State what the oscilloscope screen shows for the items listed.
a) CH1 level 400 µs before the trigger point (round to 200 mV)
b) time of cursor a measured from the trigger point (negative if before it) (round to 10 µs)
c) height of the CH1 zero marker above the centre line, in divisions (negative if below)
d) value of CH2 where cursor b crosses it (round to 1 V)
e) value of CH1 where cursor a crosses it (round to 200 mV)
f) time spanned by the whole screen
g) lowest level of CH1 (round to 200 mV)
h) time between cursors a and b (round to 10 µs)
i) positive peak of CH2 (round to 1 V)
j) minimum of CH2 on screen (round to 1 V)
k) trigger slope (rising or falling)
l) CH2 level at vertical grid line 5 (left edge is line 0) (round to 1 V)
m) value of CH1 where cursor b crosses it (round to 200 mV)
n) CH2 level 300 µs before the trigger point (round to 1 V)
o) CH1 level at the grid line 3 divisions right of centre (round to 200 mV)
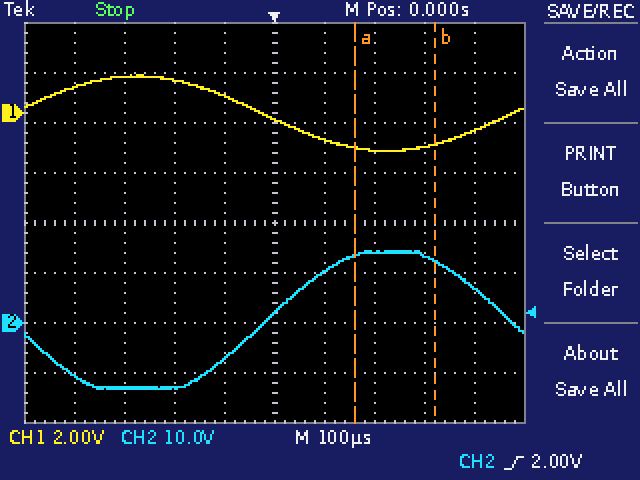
1.0 V
+160 µs
+2.2 div
12 V
-1.4 V
1 ms
-1.6 V
160 µs
14 V
-13 V
rising
2 V
-1.2 V
-13 V
-1.4 V
